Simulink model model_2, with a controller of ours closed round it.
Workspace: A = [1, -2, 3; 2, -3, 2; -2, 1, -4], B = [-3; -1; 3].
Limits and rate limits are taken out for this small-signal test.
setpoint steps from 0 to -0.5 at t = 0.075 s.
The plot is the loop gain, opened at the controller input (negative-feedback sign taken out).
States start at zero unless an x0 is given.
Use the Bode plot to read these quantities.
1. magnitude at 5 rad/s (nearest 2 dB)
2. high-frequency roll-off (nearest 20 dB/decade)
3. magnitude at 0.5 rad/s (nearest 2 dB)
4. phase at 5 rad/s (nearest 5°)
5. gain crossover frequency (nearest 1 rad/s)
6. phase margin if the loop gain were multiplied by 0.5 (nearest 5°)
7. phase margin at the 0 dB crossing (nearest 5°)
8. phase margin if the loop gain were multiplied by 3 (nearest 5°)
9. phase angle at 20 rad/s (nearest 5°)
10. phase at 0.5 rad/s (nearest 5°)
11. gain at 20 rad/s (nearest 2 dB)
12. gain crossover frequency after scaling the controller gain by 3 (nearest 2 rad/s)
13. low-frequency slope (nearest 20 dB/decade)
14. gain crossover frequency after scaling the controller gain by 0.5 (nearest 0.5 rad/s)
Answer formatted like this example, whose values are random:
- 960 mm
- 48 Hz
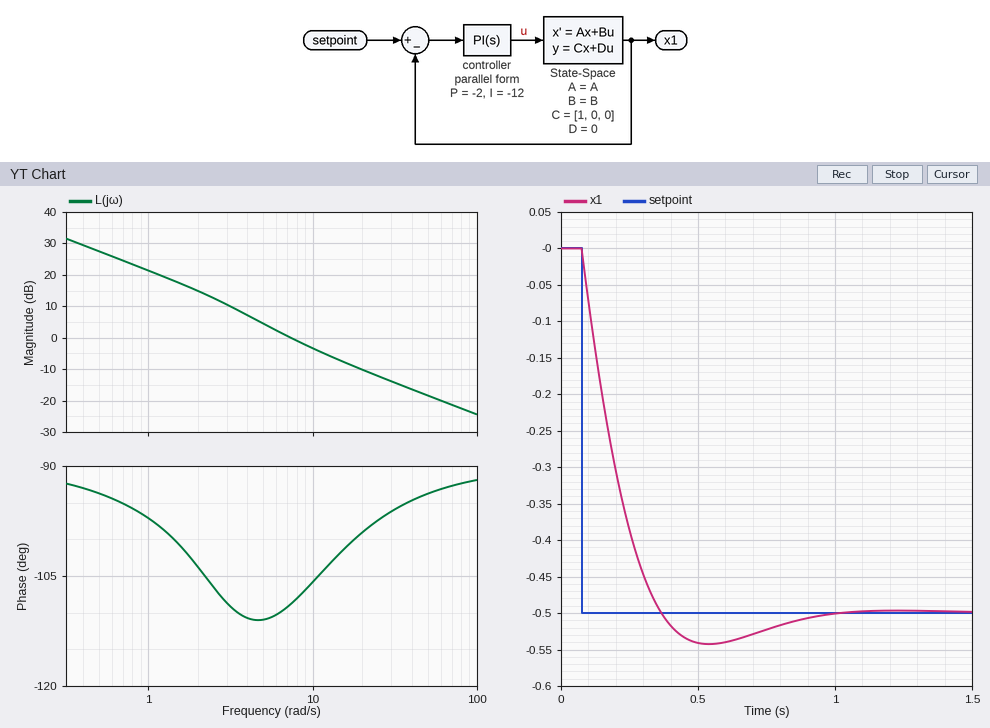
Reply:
- 4 dB
- -20 dB/decade
- 28 dB
- -110°
- 7 rad/s
- 70°
- 70°
- 80°
- -100°
- -95°
- -10 dB
- 18 rad/s
- -20 dB/decade
- 4.5 rad/s
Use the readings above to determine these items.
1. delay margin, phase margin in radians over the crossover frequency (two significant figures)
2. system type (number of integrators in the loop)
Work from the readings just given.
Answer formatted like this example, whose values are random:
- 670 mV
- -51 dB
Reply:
- 0.17 s
- 1
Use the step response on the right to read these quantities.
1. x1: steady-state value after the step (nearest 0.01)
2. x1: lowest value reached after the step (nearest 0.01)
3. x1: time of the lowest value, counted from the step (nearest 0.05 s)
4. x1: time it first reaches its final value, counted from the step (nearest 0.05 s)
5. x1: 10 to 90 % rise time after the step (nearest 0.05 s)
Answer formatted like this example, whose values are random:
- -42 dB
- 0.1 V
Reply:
- -0.50
- -0.54
- 0.45 s
- 0.30 s
- 0.20 s
